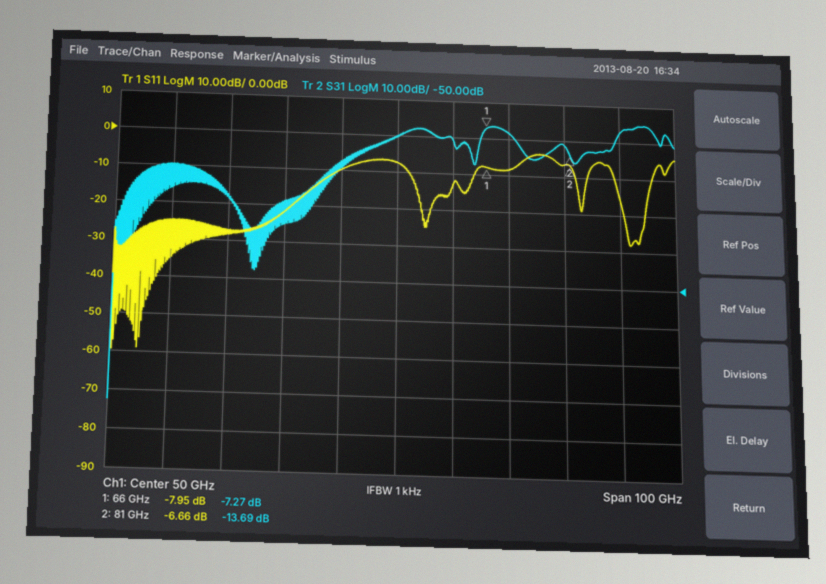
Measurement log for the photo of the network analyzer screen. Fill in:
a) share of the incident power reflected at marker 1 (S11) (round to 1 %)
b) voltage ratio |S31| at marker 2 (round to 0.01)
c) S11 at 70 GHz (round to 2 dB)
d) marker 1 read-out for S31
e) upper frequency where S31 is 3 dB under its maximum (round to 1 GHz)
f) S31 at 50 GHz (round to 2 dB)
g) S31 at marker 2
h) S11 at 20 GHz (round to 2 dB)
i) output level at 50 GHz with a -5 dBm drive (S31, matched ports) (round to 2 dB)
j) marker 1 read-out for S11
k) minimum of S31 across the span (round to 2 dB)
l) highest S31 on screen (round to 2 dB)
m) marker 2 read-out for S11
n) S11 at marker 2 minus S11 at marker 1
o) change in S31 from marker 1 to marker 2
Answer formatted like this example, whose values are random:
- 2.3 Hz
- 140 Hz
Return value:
- 16 %
- 0.21
- -8 dB
- -7.27 dB
- 97 GHz
- -10 dB
- -13.69 dB
- -28 dB
- -16 dBm
- -7.95 dB
- -82 dB
- -6 dB
- -6.66 dB
- 1.29 dB
- -6.42 dB
